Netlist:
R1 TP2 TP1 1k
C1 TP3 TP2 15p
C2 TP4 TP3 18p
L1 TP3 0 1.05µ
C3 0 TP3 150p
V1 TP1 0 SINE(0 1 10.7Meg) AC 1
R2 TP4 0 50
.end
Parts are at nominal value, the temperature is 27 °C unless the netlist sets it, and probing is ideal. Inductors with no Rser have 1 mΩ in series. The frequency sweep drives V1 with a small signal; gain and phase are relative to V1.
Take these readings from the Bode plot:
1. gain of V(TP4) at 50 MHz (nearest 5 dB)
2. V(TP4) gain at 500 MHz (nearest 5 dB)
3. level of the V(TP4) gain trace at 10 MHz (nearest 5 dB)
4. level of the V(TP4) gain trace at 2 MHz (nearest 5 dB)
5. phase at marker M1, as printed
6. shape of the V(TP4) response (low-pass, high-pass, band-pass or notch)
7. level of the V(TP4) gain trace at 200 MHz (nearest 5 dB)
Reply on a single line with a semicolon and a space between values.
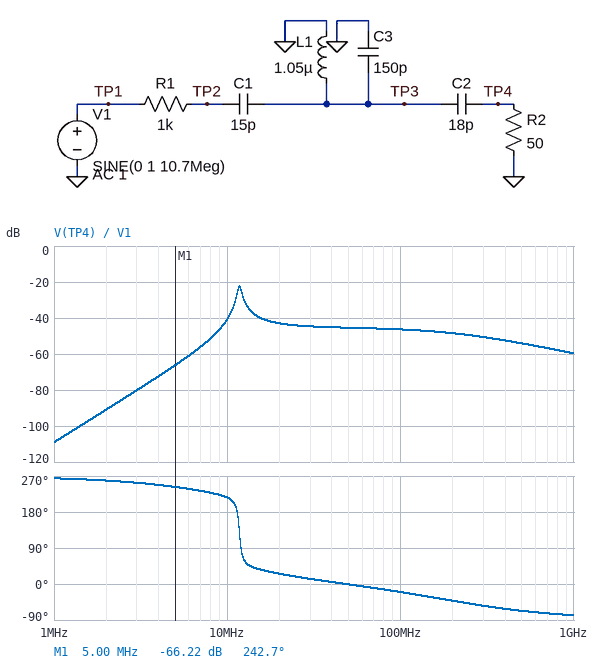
-45 dB; -55 dB; -40 dB; -90 dB; 242.7 deg; band-pass; -50 dB
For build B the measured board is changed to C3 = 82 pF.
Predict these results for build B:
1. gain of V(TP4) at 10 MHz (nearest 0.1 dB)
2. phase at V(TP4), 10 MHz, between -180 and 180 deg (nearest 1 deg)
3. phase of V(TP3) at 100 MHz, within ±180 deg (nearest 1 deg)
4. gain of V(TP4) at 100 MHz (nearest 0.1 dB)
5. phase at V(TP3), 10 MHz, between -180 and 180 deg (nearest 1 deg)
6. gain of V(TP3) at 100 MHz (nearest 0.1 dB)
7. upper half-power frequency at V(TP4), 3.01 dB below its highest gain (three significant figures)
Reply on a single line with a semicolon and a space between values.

-46.7 dB; -140 deg; -78 deg; -41.6 dB; 133 deg; -35.5 dB; 15.9 MHz
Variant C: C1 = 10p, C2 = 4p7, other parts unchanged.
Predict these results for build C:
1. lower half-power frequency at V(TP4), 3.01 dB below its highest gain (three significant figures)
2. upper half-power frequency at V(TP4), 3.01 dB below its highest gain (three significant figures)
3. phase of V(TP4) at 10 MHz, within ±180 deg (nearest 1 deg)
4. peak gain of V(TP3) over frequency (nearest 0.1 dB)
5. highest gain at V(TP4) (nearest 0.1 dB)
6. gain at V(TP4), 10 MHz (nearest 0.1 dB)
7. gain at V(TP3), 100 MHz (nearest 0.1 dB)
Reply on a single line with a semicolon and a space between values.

12.1 MHz; 12.4 MHz; -126 deg; 4.1 dB; -30.7 dB; -56.1 dB; -39.7 dB
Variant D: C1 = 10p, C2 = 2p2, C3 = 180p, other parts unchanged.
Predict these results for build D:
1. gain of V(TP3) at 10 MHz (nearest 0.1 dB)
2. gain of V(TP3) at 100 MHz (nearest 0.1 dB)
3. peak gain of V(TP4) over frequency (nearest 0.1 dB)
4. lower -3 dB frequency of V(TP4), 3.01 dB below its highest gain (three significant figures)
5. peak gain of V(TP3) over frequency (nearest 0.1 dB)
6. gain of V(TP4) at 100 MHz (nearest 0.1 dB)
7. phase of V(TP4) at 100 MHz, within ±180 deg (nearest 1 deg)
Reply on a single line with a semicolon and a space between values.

-15.8 dB; -41.2 dB; -37.4 dB; 11.2 MHz; 4.7 dB; -64.4 dB; 6 deg
